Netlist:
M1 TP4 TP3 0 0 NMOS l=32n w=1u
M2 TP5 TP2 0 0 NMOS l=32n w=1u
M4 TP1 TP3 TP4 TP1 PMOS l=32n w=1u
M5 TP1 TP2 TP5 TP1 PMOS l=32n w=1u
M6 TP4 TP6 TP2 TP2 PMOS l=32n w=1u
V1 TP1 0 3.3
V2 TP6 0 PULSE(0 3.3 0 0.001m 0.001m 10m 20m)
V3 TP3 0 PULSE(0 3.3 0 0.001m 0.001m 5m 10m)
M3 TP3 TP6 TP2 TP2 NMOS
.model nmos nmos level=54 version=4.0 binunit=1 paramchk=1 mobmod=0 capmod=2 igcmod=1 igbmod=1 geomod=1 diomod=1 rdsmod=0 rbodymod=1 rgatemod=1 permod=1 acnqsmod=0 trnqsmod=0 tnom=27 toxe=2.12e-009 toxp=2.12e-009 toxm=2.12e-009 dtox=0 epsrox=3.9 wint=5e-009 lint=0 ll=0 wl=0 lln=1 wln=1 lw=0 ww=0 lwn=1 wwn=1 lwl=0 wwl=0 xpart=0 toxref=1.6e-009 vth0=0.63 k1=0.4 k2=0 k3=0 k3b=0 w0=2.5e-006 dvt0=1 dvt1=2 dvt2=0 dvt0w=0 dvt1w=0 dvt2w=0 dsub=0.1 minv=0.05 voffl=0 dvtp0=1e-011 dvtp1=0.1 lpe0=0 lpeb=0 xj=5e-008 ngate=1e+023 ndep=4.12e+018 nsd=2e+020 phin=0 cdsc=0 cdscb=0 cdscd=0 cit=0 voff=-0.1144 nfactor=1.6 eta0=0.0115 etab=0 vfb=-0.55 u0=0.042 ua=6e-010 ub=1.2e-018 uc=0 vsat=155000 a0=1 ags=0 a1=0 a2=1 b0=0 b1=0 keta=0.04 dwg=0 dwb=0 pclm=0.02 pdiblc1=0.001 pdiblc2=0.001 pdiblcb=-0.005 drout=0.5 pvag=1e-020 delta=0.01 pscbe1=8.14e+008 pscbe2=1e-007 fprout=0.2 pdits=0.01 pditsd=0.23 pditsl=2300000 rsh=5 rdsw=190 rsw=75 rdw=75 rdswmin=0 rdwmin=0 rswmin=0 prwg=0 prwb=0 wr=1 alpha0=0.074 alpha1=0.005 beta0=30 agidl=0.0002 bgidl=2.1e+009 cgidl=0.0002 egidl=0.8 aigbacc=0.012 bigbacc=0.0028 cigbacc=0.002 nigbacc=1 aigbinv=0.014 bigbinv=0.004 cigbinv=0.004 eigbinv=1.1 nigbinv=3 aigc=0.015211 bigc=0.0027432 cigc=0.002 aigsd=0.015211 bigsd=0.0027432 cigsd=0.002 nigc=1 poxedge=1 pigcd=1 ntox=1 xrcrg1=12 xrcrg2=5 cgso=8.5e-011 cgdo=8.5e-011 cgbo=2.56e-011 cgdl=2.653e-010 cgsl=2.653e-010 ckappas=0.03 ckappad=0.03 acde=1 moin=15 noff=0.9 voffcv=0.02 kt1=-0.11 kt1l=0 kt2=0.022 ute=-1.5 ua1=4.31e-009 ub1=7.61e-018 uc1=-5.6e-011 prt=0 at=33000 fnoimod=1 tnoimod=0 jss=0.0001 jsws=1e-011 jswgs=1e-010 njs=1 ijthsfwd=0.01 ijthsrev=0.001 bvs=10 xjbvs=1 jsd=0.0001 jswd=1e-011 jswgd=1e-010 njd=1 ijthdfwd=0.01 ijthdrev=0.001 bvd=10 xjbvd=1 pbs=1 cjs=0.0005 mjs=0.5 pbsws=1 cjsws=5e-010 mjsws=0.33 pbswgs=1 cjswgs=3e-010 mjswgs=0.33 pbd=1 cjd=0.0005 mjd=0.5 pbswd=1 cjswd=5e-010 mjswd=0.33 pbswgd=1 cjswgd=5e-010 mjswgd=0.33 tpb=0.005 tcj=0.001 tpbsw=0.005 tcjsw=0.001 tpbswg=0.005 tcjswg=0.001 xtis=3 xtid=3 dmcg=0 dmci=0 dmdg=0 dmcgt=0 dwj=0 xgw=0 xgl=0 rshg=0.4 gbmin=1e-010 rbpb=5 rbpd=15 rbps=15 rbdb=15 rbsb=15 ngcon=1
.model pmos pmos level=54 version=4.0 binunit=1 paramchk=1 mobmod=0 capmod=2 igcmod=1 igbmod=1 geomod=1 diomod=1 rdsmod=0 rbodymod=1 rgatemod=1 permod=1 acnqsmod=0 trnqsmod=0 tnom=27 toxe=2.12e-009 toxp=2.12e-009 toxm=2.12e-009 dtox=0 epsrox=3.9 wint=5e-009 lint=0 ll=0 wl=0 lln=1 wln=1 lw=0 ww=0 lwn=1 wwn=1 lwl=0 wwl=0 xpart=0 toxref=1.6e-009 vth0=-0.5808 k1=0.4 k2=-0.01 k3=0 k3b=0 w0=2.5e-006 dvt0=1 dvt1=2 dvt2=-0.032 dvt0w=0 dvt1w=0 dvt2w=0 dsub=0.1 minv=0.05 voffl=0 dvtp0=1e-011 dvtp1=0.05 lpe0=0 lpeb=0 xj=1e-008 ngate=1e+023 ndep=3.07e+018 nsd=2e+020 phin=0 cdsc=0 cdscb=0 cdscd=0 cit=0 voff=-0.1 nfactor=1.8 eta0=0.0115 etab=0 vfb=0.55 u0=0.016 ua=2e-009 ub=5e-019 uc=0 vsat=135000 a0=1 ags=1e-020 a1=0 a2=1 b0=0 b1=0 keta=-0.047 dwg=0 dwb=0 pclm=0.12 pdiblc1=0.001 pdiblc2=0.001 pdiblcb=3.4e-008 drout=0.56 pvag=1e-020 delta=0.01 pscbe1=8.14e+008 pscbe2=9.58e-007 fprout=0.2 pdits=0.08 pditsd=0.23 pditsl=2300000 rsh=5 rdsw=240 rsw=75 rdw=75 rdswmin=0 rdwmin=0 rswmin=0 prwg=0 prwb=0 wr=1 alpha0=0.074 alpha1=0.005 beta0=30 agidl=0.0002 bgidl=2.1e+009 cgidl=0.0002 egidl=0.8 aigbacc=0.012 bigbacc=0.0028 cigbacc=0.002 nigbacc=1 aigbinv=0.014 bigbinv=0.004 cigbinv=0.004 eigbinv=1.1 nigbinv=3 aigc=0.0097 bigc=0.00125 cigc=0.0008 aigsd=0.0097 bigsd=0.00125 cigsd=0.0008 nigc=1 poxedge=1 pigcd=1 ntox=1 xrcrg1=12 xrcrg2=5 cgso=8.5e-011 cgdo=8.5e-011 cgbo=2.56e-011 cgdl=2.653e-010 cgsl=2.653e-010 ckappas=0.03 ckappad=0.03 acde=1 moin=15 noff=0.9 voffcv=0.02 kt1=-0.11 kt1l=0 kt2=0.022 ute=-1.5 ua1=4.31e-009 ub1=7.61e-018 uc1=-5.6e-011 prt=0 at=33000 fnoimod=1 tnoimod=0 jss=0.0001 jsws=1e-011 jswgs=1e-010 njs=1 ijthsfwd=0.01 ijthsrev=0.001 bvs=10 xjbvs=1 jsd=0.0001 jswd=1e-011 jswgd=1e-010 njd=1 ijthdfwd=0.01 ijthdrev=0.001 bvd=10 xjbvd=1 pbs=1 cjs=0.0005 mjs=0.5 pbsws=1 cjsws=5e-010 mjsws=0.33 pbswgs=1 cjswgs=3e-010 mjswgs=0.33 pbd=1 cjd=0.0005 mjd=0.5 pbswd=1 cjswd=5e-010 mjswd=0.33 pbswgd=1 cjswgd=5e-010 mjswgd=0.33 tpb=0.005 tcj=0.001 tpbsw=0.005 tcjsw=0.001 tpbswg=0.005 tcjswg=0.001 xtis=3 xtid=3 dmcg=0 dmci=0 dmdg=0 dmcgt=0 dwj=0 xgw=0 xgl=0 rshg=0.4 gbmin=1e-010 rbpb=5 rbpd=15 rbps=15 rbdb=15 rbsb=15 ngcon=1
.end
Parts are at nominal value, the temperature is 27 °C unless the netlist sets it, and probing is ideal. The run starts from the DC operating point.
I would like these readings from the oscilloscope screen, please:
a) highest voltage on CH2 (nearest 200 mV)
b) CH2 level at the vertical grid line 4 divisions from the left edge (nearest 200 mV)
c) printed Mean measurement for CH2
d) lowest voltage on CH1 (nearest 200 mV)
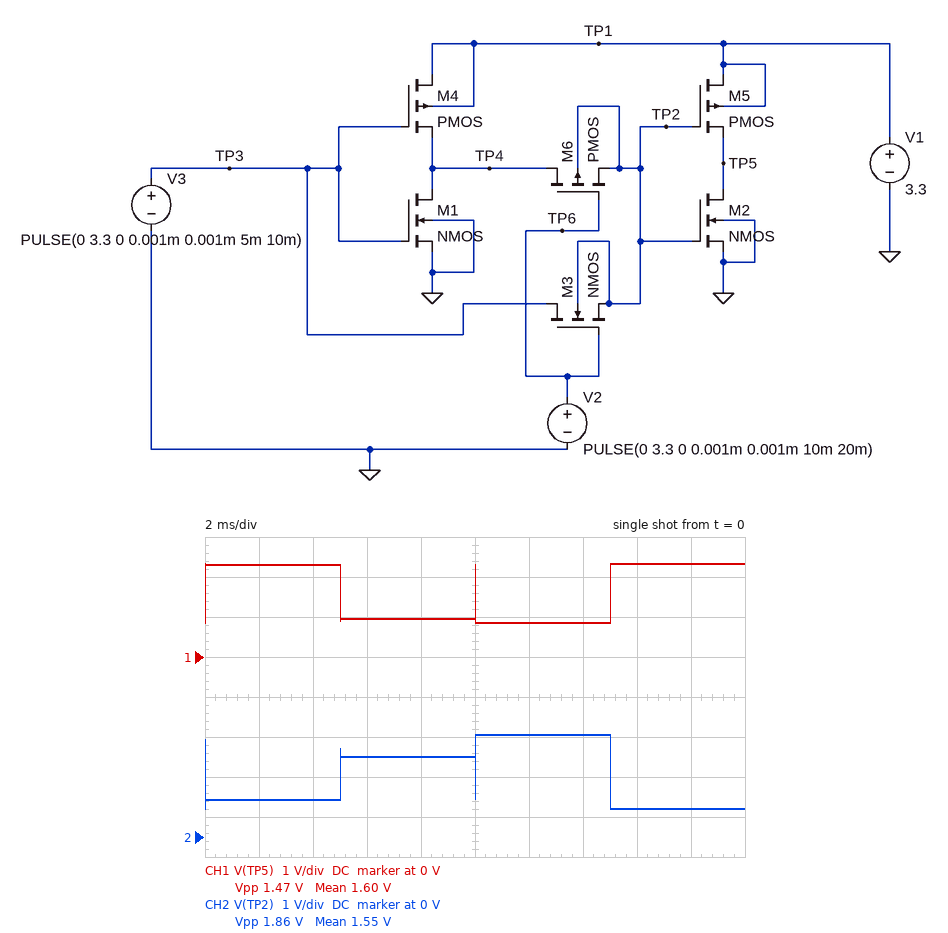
2.6 V
2.0 V
1.55 V
800 mV
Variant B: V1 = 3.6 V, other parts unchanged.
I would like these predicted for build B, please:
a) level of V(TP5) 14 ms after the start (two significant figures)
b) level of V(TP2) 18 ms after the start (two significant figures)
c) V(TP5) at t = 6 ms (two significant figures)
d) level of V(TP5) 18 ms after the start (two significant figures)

1.1 V
700 mV
1.2 V
2.4 V
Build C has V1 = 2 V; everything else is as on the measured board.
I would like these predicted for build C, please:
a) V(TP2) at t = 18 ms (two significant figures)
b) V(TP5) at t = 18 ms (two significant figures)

660 mV
1.8 V
